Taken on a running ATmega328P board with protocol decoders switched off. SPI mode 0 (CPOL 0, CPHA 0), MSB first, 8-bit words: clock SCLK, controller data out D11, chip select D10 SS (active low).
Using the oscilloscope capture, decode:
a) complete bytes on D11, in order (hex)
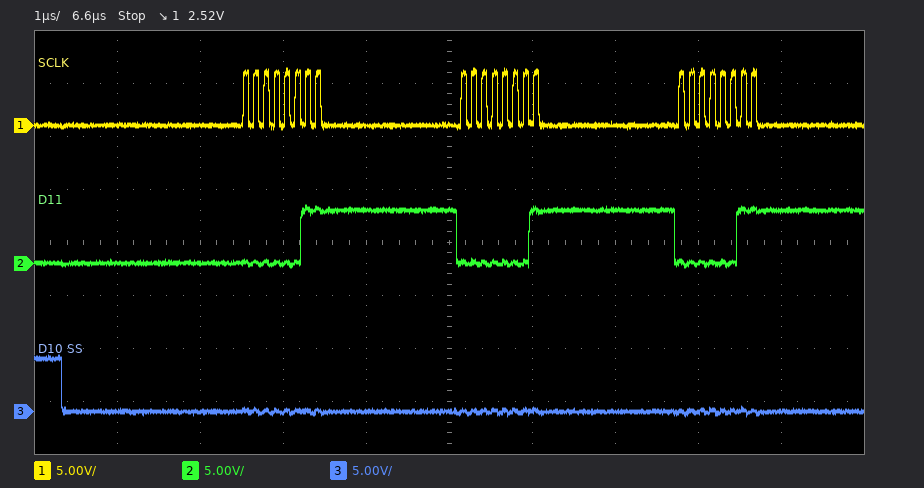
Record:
03 01 03
